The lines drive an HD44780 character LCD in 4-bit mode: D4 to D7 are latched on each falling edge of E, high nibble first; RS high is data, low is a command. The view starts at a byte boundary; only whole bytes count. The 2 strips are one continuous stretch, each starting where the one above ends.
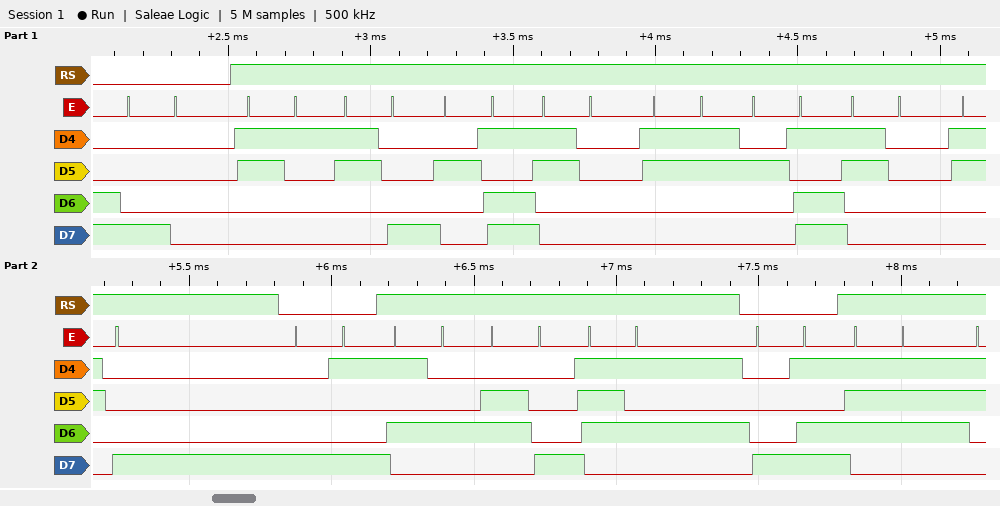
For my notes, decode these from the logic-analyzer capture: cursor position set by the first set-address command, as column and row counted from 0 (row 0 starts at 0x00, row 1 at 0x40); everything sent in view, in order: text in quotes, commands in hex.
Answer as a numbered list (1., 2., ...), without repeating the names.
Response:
1. column 0, row 0
2. 0x80 "18-03-08" 0x89 "Thu" 0x8D "w"
